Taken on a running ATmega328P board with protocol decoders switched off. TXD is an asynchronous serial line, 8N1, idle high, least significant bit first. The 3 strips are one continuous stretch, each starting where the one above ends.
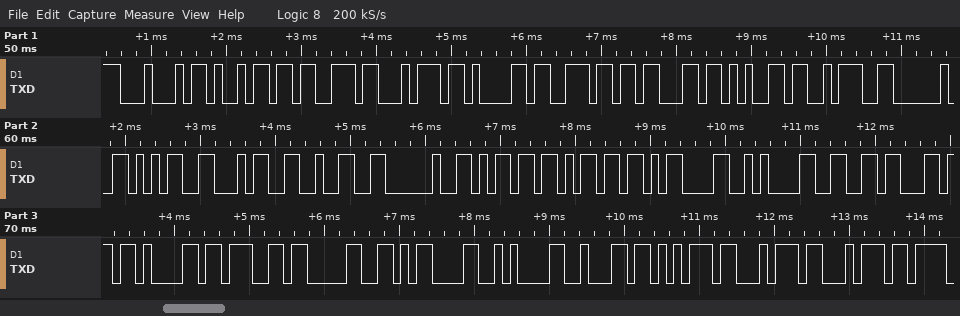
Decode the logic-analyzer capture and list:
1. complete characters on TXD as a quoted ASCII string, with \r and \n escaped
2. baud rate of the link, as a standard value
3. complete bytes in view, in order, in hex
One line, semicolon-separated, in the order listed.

"Distance: 542 mm\r\nflag0\r\nbutt"; 9600 baud; 44 69 73 74 61 6E 63 65 3A 20 35 34 32 20 6D 6D 0D 0A 66 6C 61 67 30 0D 0A 62 75 74 74
